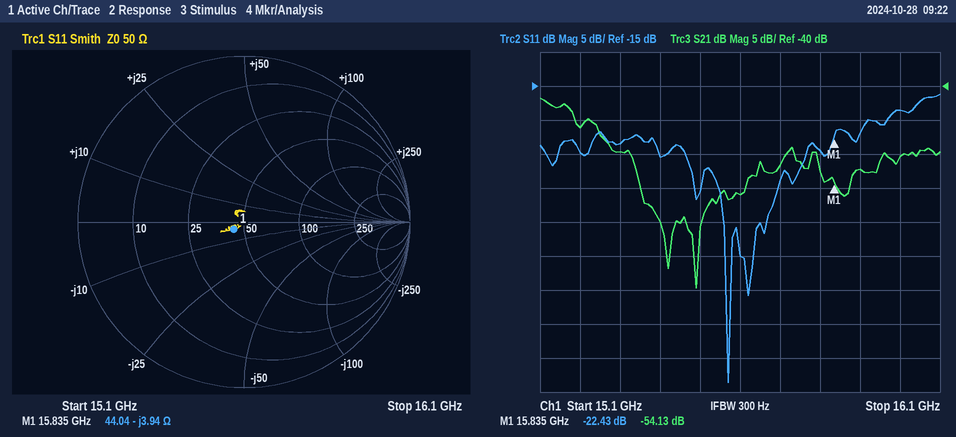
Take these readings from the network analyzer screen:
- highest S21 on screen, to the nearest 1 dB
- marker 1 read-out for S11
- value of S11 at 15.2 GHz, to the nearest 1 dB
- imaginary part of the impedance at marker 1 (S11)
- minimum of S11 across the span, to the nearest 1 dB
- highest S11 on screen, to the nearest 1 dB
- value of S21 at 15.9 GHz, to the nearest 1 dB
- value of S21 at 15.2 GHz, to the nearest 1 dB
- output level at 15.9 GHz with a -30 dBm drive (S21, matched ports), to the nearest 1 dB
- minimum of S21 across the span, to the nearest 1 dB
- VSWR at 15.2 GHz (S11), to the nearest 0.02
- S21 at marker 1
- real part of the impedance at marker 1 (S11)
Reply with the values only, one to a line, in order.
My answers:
-42 dB
-22.43 dB
-25 dB
-3.94 Ω
-59 dB
-16 dB
-52 dB
-46 dB
-82 dBm
-70 dB
1.12
-54.13 dB
44.04 Ω
